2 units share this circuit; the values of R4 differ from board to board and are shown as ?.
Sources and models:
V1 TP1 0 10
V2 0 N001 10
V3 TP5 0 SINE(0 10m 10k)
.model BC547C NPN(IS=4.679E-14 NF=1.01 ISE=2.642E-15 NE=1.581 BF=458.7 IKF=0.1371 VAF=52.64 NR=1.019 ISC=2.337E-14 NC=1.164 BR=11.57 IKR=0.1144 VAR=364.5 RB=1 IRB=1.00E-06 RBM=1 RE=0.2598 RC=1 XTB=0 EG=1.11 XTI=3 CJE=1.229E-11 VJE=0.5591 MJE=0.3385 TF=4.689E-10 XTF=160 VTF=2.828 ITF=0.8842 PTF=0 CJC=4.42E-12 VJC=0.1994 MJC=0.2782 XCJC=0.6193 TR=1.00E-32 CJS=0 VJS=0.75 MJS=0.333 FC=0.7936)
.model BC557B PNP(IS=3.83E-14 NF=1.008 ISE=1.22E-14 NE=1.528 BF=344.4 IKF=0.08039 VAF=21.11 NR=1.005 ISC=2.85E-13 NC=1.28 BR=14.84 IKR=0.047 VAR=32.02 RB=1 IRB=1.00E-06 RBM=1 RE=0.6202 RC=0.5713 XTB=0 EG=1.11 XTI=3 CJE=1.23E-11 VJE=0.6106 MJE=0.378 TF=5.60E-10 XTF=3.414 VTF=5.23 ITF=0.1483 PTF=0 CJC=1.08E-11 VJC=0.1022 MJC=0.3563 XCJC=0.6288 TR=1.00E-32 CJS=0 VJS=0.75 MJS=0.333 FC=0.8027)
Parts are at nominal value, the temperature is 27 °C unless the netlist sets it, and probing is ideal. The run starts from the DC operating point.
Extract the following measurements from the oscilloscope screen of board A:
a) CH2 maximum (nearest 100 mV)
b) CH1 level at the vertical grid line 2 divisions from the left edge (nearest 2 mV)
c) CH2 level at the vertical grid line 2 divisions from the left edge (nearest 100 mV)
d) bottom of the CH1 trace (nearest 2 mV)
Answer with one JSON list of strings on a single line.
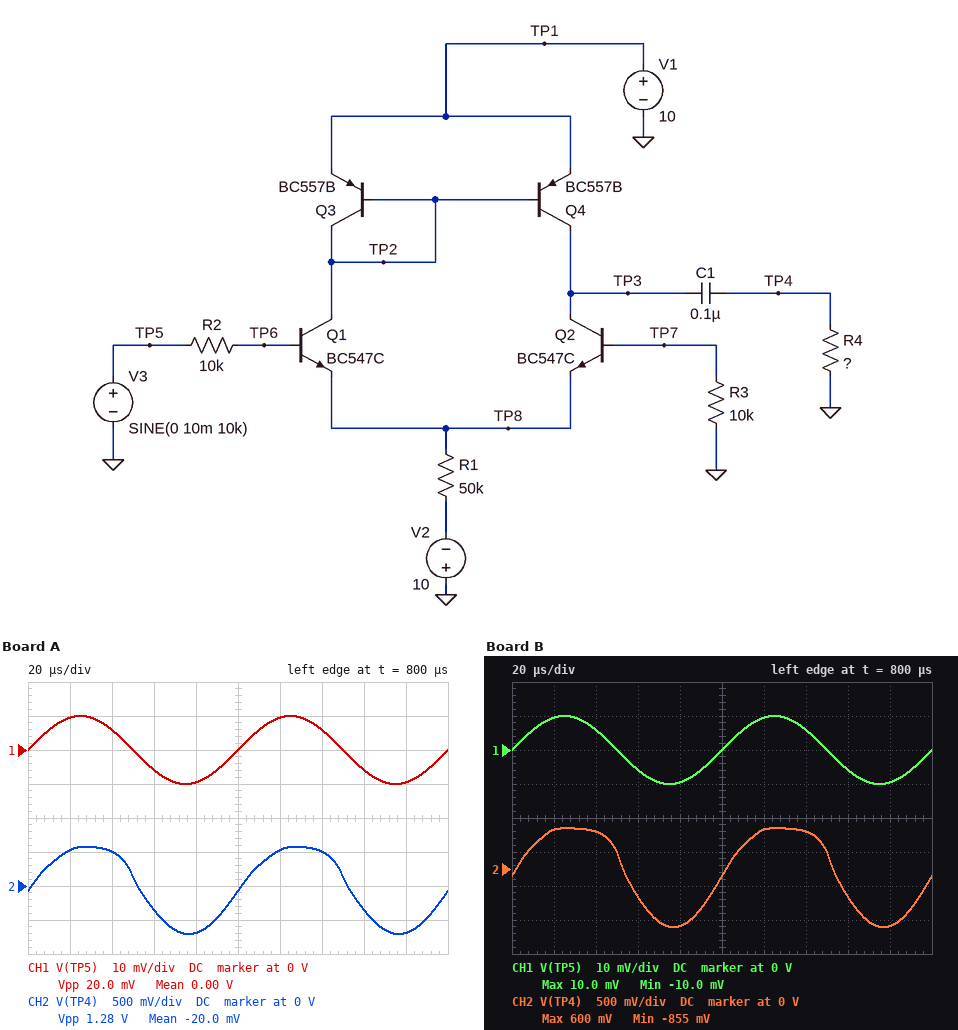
["600 mV", "6 mV", "500 mV", "-10 mV"]
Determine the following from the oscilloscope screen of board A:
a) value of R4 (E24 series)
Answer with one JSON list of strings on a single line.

["24 kΩ"]
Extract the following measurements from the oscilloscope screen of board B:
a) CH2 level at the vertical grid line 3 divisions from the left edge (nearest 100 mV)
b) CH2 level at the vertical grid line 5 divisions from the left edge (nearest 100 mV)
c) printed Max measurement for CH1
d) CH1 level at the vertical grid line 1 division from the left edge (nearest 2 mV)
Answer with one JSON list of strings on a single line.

["-400 mV", "-100 mV", "10.0 mV", "10 mV"]
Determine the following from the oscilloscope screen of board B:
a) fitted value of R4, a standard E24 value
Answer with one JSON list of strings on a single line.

["30 kΩ"]
